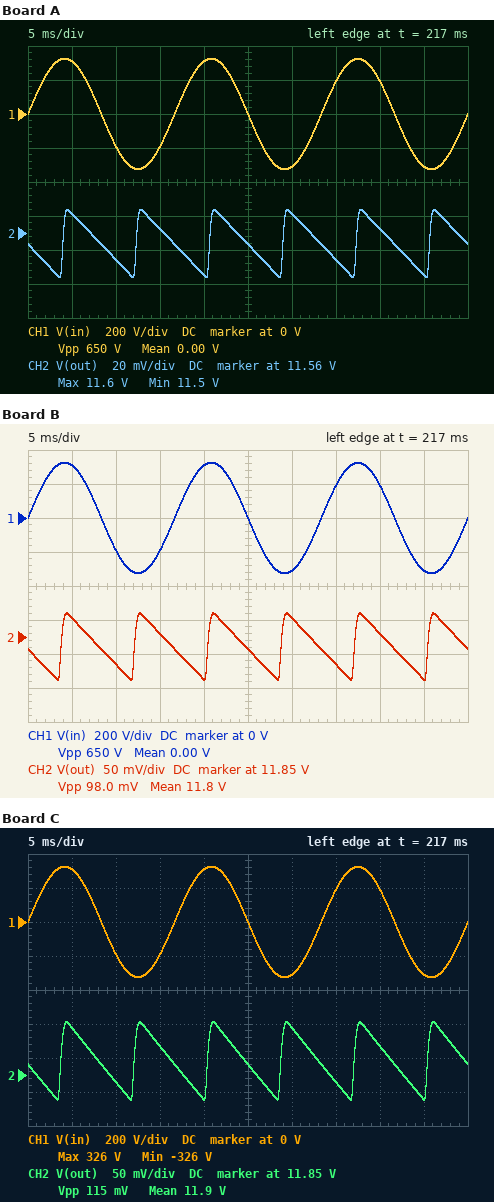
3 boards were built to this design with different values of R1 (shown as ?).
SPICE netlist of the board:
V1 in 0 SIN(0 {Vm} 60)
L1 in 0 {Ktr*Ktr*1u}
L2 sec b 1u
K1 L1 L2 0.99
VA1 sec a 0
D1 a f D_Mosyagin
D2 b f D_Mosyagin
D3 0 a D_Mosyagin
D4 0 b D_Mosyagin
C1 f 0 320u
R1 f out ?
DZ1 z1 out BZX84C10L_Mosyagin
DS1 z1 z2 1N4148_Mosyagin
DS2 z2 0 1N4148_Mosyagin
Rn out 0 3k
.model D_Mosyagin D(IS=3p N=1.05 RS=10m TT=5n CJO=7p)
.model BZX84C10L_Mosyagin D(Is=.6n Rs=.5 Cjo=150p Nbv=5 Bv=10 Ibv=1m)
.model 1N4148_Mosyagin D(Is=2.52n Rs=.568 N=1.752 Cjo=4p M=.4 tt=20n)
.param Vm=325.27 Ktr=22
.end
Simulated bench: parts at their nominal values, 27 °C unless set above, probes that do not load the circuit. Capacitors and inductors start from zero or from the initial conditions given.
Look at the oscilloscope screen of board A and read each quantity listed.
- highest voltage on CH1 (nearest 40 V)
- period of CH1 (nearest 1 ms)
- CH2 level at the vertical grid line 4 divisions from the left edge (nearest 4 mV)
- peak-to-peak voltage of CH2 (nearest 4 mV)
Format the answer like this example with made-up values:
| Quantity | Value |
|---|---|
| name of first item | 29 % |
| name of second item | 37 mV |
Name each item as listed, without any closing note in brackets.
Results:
| Quantity | Value |
|---|---|
| highest voltage on CH1 | 320 V |
| period of CH1 | 17 ms |
| CH2 level at the vertical grid line 4 divisions from the left edge | 11.536 V |
| peak-to-peak voltage of CH2 | 40 mV |
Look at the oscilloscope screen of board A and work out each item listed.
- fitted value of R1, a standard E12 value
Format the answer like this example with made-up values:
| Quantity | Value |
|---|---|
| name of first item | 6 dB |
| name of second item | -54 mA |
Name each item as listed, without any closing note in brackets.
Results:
| Quantity | Value |
|---|---|
| fitted value of R1, a standard E12 value | 180 Ω |
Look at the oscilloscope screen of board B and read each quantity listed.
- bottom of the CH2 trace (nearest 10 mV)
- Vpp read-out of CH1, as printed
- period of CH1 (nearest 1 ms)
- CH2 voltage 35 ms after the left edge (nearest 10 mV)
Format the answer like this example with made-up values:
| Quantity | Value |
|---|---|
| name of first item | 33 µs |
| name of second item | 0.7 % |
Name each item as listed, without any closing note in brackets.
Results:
| Quantity | Value |
|---|---|
| bottom of the CH2 trace | 11.79 V |
| Vpp read-out of CH1, as printed | 650 V |
| period of CH1 | 17 ms |
| CH2 voltage 35 ms after the left edge | 11.81 V |
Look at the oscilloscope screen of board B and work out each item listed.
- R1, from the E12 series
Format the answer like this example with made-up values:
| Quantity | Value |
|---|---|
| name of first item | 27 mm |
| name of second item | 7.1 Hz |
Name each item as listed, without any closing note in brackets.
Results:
| Quantity | Value |
|---|---|
| R1, from the E12 series | 56 Ω |
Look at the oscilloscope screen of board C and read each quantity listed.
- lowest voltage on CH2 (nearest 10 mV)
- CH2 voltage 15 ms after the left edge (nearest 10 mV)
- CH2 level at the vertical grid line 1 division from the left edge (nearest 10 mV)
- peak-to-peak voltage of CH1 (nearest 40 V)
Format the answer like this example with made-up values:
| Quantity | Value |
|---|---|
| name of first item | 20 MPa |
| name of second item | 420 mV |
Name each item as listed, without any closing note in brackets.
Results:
| Quantity | Value |
|---|---|
| lowest voltage on CH2 | 11.81 V |
| CH2 voltage 15 ms after the left edge | 11.89 V |
| CH2 level at the vertical grid line 1 division from the left edge | 11.92 V |
| peak-to-peak voltage of CH1 | 640 V |
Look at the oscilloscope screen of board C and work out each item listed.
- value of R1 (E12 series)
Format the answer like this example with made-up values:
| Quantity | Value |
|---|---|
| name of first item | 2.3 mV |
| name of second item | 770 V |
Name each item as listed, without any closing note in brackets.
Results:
| Quantity | Value |
|---|---|
| value of R1 | 47 Ω |
